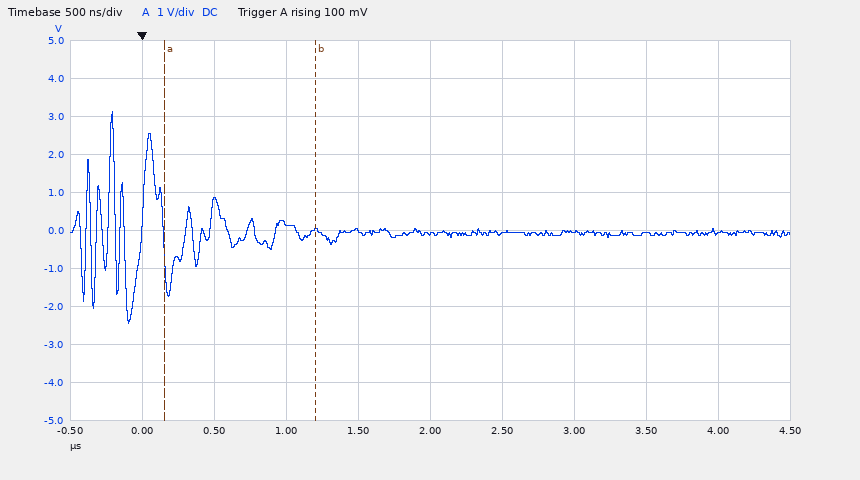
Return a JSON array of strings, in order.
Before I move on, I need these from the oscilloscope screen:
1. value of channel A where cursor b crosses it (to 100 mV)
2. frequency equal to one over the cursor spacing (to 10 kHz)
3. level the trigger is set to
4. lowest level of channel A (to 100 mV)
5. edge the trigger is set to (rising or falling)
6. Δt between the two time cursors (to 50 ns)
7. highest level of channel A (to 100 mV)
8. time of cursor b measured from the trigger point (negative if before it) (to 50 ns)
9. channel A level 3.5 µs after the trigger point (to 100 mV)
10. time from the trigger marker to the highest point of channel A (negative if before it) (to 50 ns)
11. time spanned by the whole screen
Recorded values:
["0.0 V", "950 kHz", "100 mV", "-2.4 V", "rising", "1.05 µs", "3.1 V", "+1.20 µs", "-100 mV", "-200 ns", "5 µs"]
